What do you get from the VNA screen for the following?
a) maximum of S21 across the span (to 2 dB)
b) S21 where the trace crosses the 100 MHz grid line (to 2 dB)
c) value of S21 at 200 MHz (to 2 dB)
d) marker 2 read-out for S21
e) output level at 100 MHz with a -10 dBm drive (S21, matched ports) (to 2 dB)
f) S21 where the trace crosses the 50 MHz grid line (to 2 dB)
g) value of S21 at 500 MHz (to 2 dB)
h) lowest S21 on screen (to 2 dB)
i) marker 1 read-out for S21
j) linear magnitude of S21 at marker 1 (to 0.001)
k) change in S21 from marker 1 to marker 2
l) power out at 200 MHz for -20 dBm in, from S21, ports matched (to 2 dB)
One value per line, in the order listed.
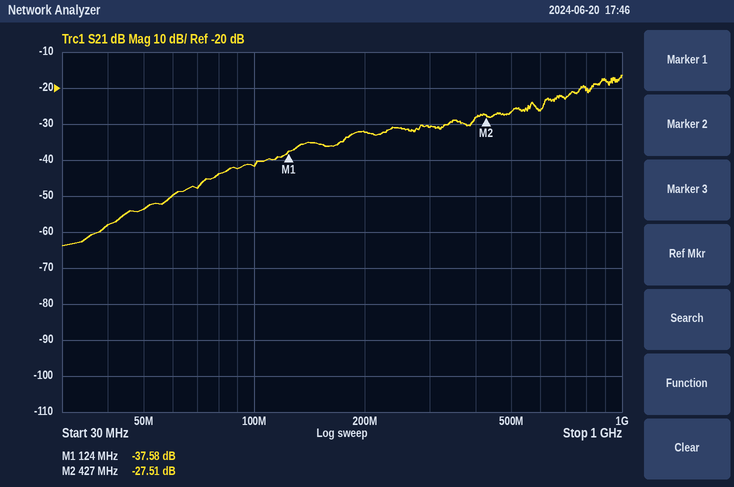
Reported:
-16 dB
-42 dB
-32 dB
-27.51 dB
-52 dBm
-54 dB
-26 dB
-64 dB
-37.58 dB
0.013
10.07 dB
-52 dBm
